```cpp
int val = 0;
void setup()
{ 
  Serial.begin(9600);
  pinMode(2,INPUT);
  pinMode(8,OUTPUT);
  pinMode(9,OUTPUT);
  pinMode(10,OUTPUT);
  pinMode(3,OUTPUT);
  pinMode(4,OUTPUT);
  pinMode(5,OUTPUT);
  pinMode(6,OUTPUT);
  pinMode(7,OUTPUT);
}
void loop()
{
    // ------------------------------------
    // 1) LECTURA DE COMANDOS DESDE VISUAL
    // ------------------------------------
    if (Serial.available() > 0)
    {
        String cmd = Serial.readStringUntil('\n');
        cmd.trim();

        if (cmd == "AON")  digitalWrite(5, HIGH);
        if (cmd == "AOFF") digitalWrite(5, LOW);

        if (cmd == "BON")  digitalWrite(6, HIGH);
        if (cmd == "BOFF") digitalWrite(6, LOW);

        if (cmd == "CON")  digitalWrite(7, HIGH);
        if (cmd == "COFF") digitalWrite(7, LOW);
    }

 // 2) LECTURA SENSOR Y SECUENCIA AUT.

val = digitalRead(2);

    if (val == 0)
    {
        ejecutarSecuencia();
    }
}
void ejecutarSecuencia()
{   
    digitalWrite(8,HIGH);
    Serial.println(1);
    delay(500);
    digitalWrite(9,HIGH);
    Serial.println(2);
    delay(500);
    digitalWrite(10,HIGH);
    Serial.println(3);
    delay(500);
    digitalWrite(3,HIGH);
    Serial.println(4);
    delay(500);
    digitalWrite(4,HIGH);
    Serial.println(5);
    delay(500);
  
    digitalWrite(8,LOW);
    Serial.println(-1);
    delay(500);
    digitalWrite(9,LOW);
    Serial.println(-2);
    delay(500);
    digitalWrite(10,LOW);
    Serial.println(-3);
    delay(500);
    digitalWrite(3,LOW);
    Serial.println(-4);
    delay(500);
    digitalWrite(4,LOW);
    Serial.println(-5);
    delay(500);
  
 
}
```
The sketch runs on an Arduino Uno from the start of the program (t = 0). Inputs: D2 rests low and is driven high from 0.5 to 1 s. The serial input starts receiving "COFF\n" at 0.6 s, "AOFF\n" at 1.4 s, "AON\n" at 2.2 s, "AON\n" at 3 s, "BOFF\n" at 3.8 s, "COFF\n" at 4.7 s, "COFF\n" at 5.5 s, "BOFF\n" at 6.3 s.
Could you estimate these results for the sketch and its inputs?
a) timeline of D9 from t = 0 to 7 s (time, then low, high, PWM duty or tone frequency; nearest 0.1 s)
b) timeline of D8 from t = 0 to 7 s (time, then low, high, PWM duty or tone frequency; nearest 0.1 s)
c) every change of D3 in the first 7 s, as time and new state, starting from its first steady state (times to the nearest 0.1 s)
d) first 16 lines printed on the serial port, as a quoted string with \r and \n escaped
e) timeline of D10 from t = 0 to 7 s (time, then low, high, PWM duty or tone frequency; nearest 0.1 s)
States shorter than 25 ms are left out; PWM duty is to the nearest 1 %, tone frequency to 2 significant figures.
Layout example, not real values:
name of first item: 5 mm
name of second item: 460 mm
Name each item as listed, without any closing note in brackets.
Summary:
timeline of D9 from t = 0 to 7 s: 0 s low; 0.5 s high; 3 s low; 5.5 s high
timeline of D8 from t = 0 to 7 s: 0 s high; 2.5 s low; 5 s high
every change of D3 in the first 7 s, as time and new state, starting from its first steady state: 0 s low; 1.5 s high; 4 s low; 6.5 s high
first 16 lines printed on the serial port, as a quoted string with \r and \n escaped: "1\r\n2\r\n3\r\n4\r\n5\r\n-1\r\n-2\r\n-3\r\n-4\r\n-5\r\n1\r\n2\r\n3\r\n4\r\n5\r\n-1\r\n"
timeline of D10 from t = 0 to 7 s: 0 s low; 1 s high; 3.5 s low; 6 s high
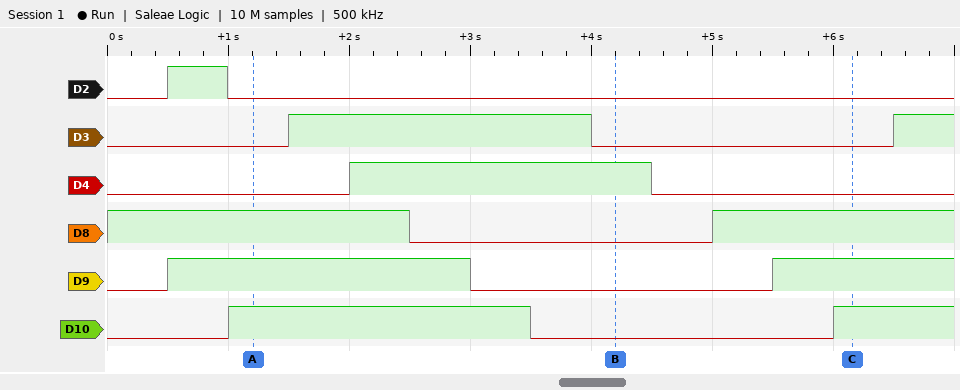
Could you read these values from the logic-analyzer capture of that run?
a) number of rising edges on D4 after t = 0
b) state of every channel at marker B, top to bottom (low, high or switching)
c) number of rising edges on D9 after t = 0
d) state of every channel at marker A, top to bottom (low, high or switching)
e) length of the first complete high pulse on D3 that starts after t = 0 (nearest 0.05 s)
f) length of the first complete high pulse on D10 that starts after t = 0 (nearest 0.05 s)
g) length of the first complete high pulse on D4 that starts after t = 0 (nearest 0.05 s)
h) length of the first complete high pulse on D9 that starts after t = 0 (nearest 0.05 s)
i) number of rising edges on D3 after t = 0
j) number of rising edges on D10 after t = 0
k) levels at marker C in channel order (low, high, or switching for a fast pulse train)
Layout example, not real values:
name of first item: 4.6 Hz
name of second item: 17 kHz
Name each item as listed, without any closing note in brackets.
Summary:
number of rising edges on D4 after t = 0: 1
state of every channel at marker B, top to bottom: D2 low, D3 low, D4 high, D8 low, D9 low, D10 low
number of rising edges on D9 after t = 0: 2
state of every channel at marker A, top to bottom: D2 low, D3 low, D4 low, D8 high, D9 high, D10 high
length of the first complete high pulse on D3 that starts after t = 0: 2.50 s
length of the first complete high pulse on D10 that starts after t = 0: 2.50 s
length of the first complete high pulse on D4 that starts after t = 0: 2.50 s
length of the first complete high pulse on D9 that starts after t = 0: 2.50 s
number of rising edges on D3 after t = 0: 2
number of rising edges on D10 after t = 0: 2
levels at marker C in channel order: D2 low, D3 low, D4 low, D8 high, D9 high, D10 high
